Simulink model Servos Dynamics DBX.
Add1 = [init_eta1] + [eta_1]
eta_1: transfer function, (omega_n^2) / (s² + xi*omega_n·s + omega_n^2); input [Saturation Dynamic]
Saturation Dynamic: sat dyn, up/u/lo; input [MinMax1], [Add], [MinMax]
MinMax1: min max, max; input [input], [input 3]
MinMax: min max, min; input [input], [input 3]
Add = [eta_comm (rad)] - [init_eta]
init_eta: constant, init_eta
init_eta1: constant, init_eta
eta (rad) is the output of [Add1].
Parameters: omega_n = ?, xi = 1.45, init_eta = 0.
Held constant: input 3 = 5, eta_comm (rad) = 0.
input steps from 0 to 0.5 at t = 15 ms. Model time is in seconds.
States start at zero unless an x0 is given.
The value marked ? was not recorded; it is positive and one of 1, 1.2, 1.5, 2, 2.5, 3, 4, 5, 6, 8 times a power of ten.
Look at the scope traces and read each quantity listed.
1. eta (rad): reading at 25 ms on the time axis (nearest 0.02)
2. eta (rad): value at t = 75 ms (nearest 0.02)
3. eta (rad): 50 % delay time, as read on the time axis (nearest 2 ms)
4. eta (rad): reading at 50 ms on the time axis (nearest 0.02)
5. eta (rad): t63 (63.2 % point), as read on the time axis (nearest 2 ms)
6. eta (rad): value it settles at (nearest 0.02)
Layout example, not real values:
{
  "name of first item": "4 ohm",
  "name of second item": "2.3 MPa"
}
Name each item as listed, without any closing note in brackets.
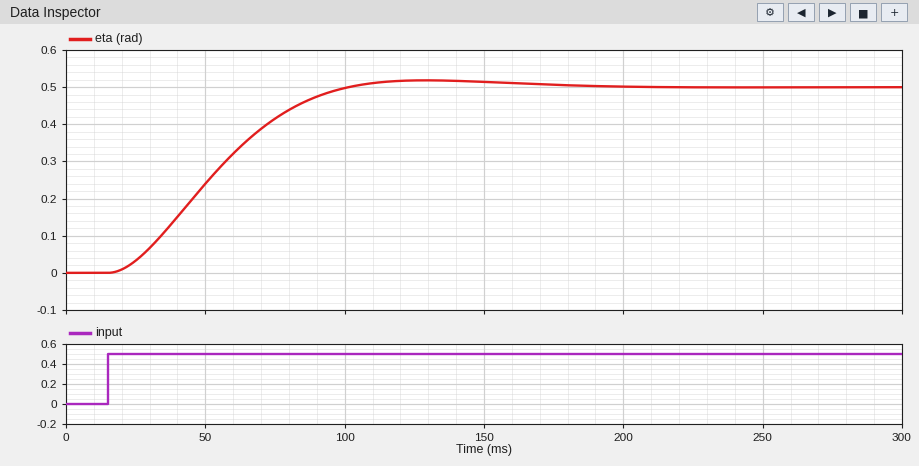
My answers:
{
  "eta (rad): reading at 25 ms on the time axis": "0.04",
  "eta (rad): value at t = 75 ms": "0.42",
  "eta (rad): 50 % delay time, as read on the time axis": "52 ms",
  "eta (rad): reading at 50 ms on the time axis": "0.24",
  "eta (rad): t63 (63.2 % point), as read on the time axis": "60 ms",
  "eta (rad): value it settles at": "0.50"
}
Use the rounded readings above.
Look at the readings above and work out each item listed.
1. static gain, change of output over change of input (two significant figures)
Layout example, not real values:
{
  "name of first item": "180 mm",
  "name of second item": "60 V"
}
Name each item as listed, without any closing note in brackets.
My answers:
{
  "static gain, change of output over change of input": "1.0"
}
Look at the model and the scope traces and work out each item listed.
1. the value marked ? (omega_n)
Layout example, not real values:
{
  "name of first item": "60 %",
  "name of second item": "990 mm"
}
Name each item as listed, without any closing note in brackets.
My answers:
{
  "the value marked ?": "40"
}
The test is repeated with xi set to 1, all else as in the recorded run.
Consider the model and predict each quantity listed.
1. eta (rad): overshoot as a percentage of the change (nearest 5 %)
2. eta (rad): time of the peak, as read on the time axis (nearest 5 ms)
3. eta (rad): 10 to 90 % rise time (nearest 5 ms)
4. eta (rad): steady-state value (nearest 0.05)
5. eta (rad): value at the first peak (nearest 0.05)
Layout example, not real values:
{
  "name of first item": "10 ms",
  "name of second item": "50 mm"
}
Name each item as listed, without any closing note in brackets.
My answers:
{
  "eta (rad): overshoot as a percentage of the change": "15 %",
  "eta (rad): time of the peak, as read on the time axis": "105 ms",
  "eta (rad): 10 to 90 % rise time": "40 ms",
  "eta (rad): steady-state value": "0.50",
  "eta (rad): value at the first peak": "0.60"
}
